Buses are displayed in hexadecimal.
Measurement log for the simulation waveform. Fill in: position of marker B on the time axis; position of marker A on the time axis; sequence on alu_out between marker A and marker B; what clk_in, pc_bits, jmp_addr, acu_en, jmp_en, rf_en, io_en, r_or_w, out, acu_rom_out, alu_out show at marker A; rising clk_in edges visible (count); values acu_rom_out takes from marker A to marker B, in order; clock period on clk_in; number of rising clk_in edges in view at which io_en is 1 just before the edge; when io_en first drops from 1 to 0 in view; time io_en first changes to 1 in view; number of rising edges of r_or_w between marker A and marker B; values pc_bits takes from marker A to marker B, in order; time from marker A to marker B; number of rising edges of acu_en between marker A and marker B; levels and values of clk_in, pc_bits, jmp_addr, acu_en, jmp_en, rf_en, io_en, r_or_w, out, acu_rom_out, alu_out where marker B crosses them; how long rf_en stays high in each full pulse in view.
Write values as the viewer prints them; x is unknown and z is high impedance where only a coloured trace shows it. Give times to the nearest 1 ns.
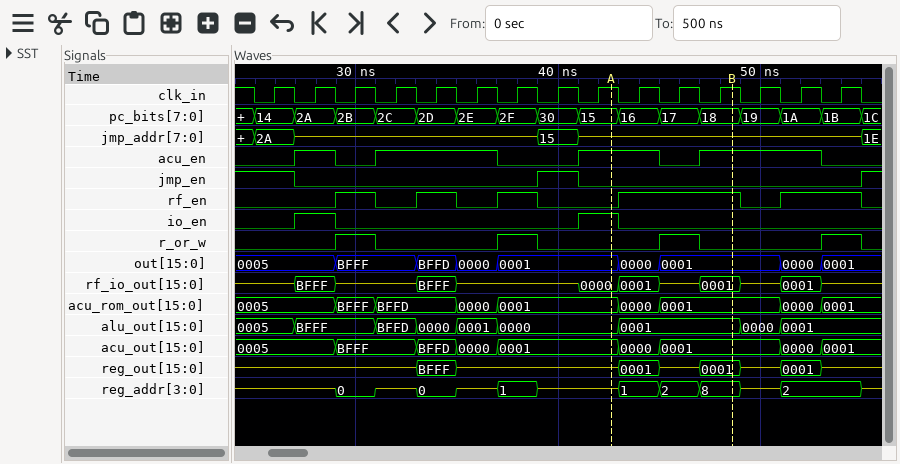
49 ns
43 ns
0000, 0001
clk_in=1, pc_bits=15, jmp_addr=z, acu_en=1, jmp_en=0, rf_en=0, io_en=1, r_or_w=0, out=0001, acu_rom_out=0001, alu_out=0000
15
0001, 0000, 0001
2 ns
2
29 ns
27 ns
1
15, 16, 17, 18
6 ns
1
clk_in=1, pc_bits=18, jmp_addr=z, acu_en=1, jmp_en=0, rf_en=1, io_en=0, r_or_w=0, out=0001, acu_rom_out=0001, alu_out=0001
2 ns, 2 ns, 2 ns, 6 ns, 4 ns
